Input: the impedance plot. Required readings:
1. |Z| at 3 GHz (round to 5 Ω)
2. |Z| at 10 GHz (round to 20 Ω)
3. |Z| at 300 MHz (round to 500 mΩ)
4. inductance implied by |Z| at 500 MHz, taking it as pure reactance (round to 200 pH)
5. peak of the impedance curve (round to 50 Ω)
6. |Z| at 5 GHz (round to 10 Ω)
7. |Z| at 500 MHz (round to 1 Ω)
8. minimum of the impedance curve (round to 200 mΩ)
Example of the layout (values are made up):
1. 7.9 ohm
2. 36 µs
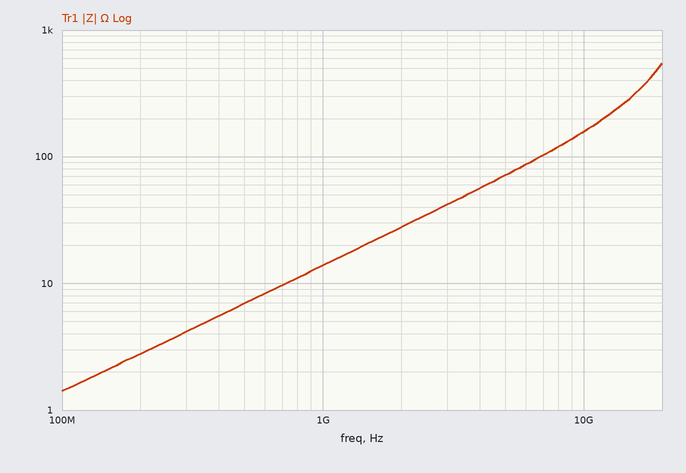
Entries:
1. 40 Ω
2. 160 Ω
3. 4.0 Ω
4. 2.2 nH
5. 550 Ω
6. 70 Ω
7. 7 Ω
8. 1.4 Ω
